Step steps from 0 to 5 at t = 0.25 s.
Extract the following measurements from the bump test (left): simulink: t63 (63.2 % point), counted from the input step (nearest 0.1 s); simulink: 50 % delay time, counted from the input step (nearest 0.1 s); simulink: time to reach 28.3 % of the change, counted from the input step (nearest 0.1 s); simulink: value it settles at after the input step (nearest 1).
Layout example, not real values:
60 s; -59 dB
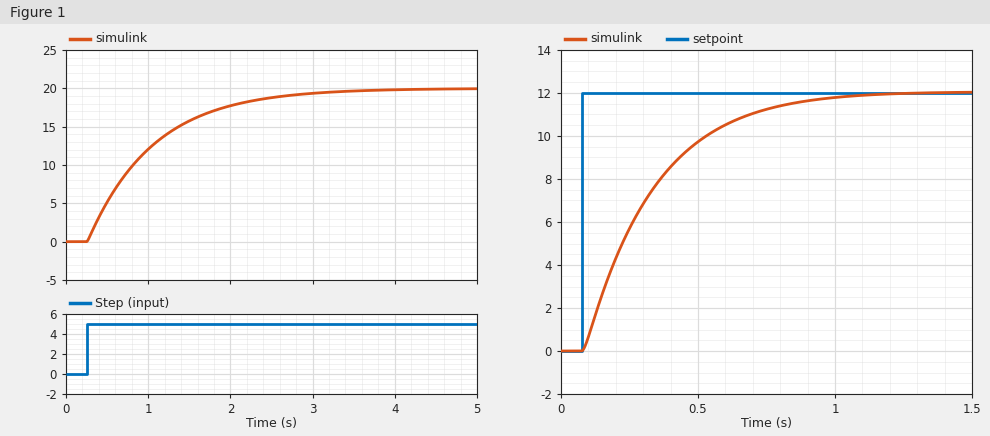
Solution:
0.8 s; 0.6 s; 0.3 s; 20
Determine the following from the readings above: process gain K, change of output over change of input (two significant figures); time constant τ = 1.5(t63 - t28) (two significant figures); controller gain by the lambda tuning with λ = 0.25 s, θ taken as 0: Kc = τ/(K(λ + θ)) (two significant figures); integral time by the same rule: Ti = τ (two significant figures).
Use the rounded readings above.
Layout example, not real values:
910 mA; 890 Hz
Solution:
4.0; 0.75 s; 0.75; 0.75 s
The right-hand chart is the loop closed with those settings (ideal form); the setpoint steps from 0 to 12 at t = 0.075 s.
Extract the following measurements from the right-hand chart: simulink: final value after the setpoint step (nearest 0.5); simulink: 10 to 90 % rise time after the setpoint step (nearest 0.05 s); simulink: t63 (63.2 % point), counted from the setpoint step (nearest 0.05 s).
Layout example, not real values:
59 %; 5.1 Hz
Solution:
12.0; 0.55 s; 0.25 s
